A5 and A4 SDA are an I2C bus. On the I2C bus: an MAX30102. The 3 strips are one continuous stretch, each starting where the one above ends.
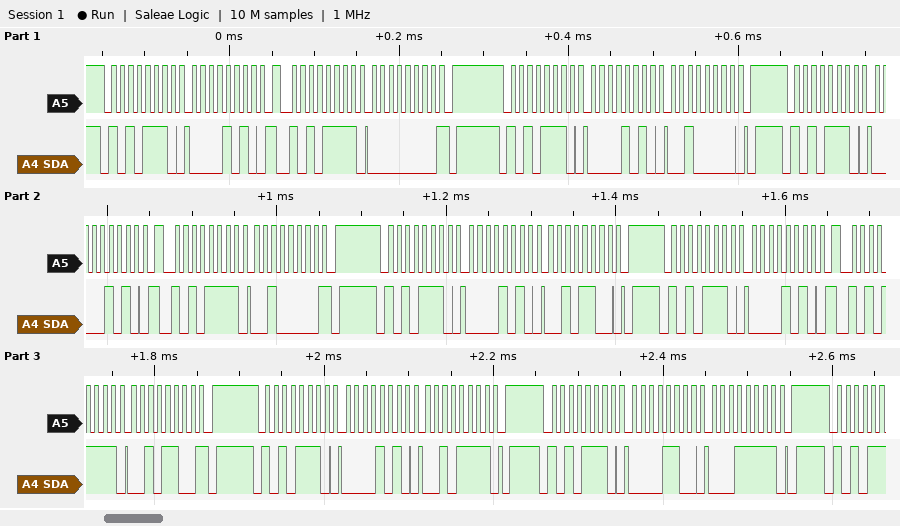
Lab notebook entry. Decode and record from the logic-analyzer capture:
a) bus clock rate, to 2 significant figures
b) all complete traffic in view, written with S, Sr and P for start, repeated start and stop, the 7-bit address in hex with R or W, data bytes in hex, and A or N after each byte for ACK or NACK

100 kHz
S 57W A 0A A Sr 57R A 00 N P S 57W A 0A A 20 A P S 57W A 0A A Sr 57R A 20 N P S 57W A 0A A 2C A P S 57W A 0A A Sr 57R A 2C N P S 57W A 0A A 2F A P S 57W A 0C A 1F A P
